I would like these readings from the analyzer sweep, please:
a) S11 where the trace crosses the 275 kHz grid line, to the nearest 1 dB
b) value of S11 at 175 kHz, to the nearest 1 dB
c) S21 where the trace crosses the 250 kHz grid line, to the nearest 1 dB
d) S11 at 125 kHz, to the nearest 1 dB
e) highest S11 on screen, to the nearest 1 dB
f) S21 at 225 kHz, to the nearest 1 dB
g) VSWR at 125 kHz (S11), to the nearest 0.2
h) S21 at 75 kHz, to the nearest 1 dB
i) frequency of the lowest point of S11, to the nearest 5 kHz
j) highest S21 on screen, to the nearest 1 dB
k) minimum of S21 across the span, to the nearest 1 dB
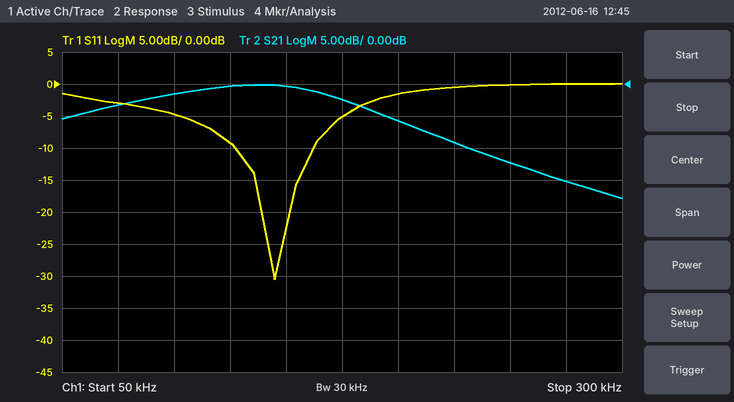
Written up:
0 dB
-5 dB
-12 dB
-9 dB
0 dB
-9 dB
2.0
-3 dB
145 kHz
0 dB
-18 dB
